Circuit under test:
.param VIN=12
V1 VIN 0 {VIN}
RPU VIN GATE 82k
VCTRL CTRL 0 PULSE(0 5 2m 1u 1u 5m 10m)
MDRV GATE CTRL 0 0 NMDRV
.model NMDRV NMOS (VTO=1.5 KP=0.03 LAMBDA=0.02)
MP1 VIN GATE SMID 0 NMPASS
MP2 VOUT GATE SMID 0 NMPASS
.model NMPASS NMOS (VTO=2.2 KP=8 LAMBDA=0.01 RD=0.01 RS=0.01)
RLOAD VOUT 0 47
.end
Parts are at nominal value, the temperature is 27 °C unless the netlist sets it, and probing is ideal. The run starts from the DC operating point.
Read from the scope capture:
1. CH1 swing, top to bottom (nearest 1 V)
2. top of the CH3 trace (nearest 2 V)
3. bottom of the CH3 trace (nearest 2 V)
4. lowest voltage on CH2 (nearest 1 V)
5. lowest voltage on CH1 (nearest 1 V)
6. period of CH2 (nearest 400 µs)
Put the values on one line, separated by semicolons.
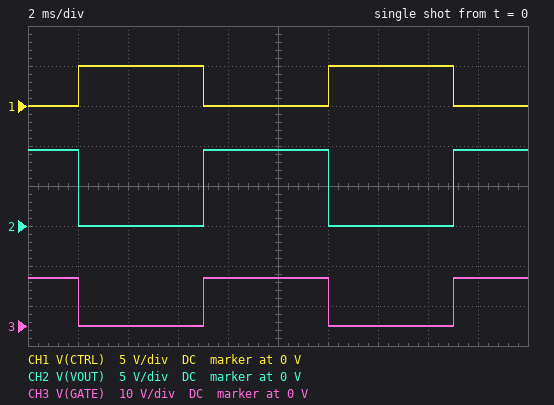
5 V; 12 V; 0 V; 0 V; 0 V; 10.0 ms
